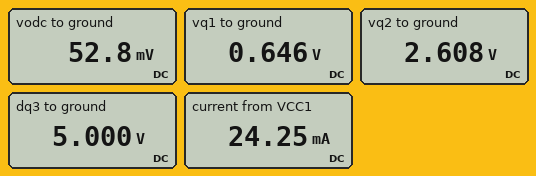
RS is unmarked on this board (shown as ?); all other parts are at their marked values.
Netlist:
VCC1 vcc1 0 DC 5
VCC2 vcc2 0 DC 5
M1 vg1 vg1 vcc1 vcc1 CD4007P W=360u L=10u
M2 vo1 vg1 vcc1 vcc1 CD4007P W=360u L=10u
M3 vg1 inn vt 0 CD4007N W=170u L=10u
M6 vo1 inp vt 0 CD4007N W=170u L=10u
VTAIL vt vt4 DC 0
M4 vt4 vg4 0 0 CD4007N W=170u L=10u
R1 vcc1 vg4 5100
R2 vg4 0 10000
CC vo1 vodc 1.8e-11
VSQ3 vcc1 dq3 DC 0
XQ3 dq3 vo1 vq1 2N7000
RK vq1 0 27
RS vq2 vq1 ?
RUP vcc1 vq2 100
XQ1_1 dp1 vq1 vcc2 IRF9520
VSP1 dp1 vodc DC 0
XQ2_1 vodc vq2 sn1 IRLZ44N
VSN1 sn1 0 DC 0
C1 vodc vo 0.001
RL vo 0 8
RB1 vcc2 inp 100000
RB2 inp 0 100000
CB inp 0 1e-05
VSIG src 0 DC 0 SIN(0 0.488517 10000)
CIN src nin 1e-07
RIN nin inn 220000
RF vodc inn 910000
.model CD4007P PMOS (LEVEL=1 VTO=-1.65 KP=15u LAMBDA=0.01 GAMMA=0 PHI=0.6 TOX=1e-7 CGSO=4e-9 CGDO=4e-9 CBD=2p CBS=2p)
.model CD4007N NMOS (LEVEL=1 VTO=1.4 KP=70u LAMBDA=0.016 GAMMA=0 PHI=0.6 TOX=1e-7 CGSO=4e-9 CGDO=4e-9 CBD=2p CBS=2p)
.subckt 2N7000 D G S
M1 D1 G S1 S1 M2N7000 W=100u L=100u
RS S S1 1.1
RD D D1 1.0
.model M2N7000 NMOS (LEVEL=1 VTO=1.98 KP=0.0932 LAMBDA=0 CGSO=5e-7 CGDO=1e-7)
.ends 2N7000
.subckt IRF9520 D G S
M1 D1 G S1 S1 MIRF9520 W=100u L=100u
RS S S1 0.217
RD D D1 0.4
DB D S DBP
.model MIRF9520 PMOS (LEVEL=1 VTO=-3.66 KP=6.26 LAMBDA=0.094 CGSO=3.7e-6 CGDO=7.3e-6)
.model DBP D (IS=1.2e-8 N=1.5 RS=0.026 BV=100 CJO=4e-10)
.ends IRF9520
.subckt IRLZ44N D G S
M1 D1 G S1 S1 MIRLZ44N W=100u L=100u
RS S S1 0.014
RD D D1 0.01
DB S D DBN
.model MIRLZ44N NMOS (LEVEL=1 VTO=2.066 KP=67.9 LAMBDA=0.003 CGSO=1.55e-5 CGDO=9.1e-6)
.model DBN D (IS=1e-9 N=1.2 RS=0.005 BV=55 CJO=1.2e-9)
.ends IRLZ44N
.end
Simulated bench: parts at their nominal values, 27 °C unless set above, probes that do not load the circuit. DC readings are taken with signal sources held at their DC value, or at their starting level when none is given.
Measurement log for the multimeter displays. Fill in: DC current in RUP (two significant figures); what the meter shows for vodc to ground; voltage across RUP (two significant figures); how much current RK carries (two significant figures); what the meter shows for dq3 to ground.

24 mA
52.8 mV
2.4 V
24 mA
5.000 V
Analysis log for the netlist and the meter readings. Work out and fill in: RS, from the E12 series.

82 Ω
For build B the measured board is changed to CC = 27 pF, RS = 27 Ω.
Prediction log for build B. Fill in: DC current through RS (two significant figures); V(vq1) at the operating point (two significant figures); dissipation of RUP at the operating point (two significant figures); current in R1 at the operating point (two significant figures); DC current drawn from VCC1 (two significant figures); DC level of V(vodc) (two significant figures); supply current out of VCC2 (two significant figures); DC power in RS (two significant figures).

29 mA
1.3 V
85 mW
330 µA
49 mA
2.5 V
7.9 mA
23 mW
